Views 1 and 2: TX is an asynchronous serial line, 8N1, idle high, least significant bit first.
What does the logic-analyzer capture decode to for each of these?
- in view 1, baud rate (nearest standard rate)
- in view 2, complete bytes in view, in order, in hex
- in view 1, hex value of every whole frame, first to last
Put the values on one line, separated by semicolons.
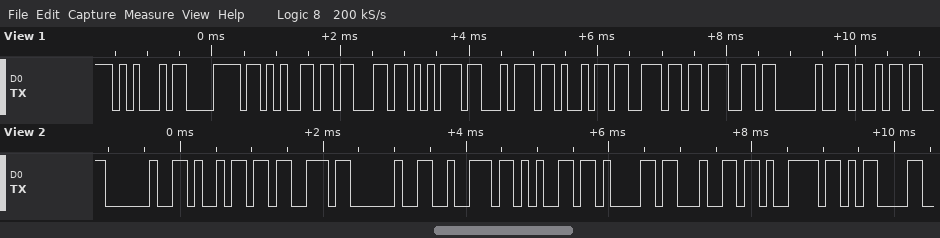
9600 baud; 0x20 0x69 0x73 0x20 0x72 0x65 0x61 0x64 0x79 0x0D; 45 78 65 63 75 74 69 6E 67 20 69
